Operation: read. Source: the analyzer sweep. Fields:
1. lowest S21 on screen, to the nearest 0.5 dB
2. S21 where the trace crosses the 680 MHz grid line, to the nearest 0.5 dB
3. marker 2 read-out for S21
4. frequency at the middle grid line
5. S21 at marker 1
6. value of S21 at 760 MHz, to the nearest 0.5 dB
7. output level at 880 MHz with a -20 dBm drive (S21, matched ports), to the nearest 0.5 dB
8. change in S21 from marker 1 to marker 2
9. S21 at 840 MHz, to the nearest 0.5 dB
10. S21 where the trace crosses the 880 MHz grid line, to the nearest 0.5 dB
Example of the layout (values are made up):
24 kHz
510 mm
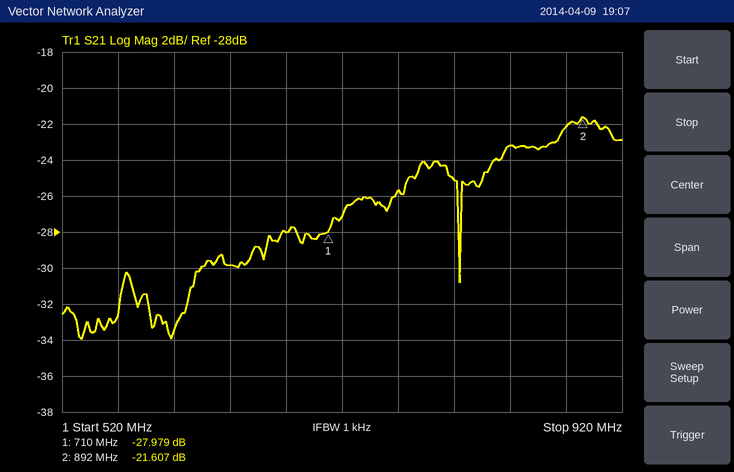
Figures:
-34.0 dB
-28.0 dB
-21.607 dB
720 MHz
-27.979 dB
-25.5 dB
-42.0 dBm
6.372 dB
-23.0 dB
-22.0 dB
